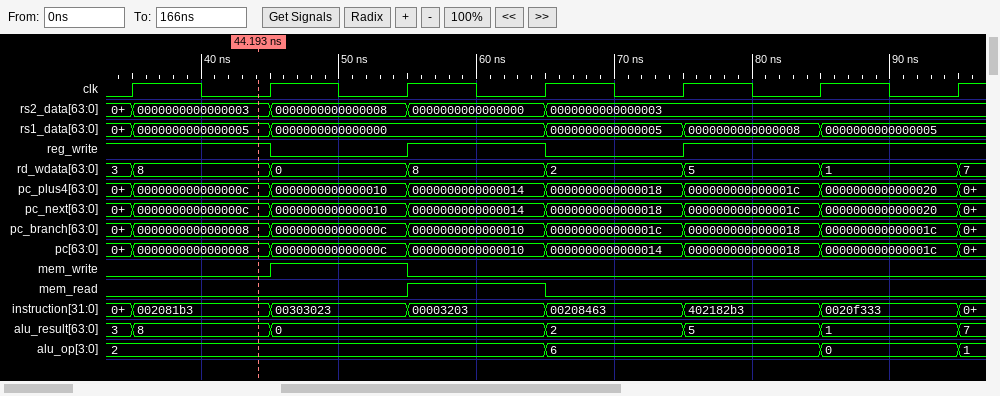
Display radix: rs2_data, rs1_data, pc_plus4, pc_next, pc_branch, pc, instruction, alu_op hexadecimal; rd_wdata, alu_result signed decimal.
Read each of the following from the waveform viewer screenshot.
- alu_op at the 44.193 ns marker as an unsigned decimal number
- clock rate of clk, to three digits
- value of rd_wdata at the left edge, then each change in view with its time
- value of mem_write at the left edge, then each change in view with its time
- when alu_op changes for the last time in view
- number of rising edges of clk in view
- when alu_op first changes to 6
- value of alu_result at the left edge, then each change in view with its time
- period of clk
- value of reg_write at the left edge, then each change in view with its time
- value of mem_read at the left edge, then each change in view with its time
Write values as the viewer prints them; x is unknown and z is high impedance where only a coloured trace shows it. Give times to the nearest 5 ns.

2
100 MHz
3, 8 at 35 ns, 0 at 45 ns, 8 at 55 ns, 2 at 65 ns, 5 at 75 ns, 1 at 85 ns, 7 at 95 ns
0, 1 at 45 ns, 0 at 55 ns
95 ns
7
65 ns
3, 8 at 35 ns, 0 at 45 ns, 2 at 65 ns, 5 at 75 ns, 1 at 85 ns, 7 at 95 ns
10 ns
1, 0 at 45 ns, 1 at 55 ns, 0 at 65 ns, 1 at 75 ns
0, 1 at 55 ns, 0 at 65 ns
